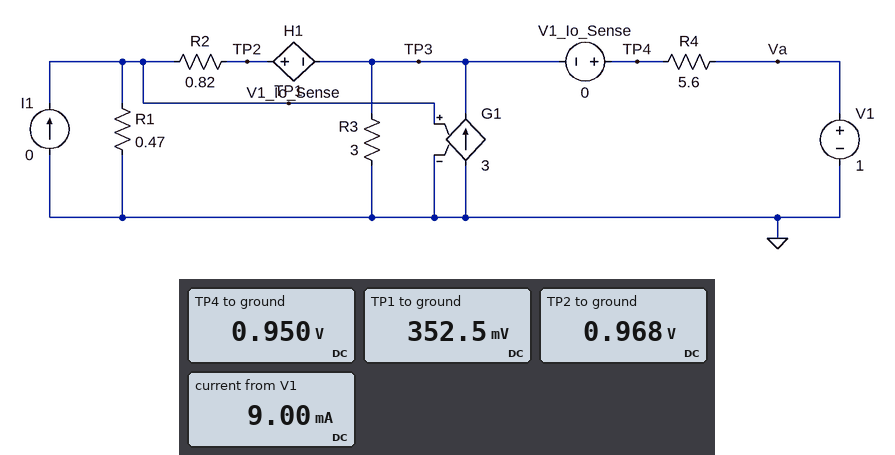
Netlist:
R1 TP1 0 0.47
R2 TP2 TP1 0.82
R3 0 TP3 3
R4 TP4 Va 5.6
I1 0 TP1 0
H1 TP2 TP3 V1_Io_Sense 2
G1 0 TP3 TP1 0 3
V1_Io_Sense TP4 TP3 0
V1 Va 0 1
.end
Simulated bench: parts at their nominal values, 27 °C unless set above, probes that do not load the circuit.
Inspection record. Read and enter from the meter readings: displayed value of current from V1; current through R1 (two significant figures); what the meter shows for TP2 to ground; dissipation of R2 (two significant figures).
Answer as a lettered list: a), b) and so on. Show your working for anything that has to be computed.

a) 9.00 mA
b) (352.5 mV) / 470 mΩ = 750 mA
c) 0.968 V
d) (968 mV - 352.5 mV)^2 / 820 mΩ = 460 mW
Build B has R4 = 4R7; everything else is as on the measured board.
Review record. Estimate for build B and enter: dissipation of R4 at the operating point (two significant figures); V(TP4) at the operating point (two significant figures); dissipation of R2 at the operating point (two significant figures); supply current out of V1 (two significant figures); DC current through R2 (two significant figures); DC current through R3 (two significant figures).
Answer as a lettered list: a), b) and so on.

a) 390 µW
b) 960 mV
c) 470 mW
d) 9.1 mA
e) 760 mA
f) 320 mA
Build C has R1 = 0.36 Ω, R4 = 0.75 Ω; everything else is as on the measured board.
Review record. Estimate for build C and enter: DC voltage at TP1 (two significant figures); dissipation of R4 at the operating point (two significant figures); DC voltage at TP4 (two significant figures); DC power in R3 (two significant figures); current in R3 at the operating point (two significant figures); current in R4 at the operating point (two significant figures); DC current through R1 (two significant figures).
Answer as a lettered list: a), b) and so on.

a) 380 mV
b) 30 mW
c) 850 mV
d) 240 mW
e) 280 mA
f) 200 mA
g) 1.1 A
